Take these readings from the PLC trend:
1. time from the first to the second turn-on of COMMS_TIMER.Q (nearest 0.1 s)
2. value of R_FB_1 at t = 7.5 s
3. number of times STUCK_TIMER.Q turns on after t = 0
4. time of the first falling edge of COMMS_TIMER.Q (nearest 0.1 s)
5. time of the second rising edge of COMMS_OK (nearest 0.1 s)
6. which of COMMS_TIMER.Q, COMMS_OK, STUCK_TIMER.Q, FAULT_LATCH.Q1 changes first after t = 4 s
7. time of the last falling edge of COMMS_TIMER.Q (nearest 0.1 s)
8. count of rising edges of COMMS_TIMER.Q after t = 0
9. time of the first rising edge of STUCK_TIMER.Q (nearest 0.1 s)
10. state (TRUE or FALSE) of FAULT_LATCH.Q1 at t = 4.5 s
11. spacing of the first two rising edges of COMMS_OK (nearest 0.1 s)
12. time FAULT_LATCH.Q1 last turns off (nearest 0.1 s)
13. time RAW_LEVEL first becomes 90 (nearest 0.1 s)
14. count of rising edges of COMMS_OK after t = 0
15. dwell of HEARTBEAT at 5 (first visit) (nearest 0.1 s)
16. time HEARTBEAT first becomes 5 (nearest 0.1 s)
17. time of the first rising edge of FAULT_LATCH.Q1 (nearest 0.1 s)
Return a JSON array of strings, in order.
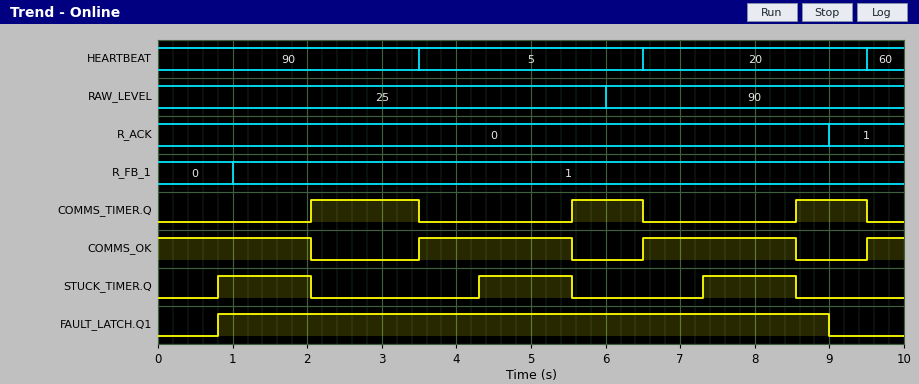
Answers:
["3.5 s", "1", "3", "3.5 s", "6.5 s", "STUCK_TIMER.Q", "9.5 s", "3", "0.8 s", "TRUE", "3.0 s", "9.0 s", "6.0 s", "3", "3.0 s", "3.5 s", "0.8 s"]
